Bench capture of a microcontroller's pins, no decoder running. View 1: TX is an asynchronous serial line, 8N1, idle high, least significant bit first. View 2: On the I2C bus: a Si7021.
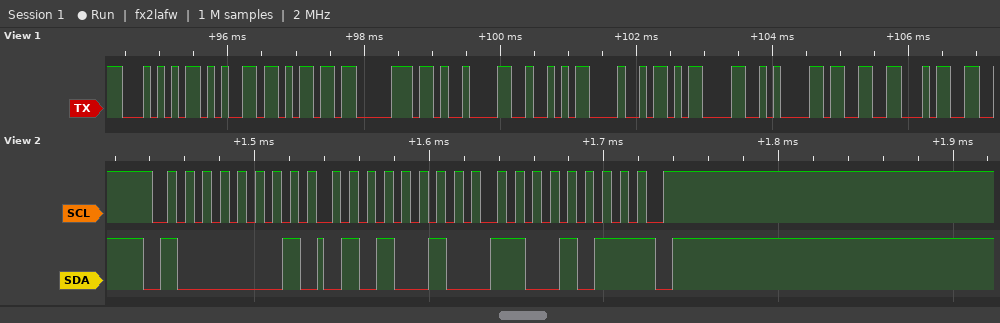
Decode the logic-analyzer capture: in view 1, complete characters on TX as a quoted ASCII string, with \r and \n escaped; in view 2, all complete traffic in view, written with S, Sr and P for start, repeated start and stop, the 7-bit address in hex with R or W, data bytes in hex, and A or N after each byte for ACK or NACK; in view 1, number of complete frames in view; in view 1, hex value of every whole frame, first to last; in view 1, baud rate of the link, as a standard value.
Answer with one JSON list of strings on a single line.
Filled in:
["\"Temp\\tRH\\r\\n34\"", "S 40R A 52 A CB N P", "11", "0x54 0x65 0x6D 0x70 0x09 0x52 0x48 0x0D 0x0A 0x33 0x34", "9600 baud"]
